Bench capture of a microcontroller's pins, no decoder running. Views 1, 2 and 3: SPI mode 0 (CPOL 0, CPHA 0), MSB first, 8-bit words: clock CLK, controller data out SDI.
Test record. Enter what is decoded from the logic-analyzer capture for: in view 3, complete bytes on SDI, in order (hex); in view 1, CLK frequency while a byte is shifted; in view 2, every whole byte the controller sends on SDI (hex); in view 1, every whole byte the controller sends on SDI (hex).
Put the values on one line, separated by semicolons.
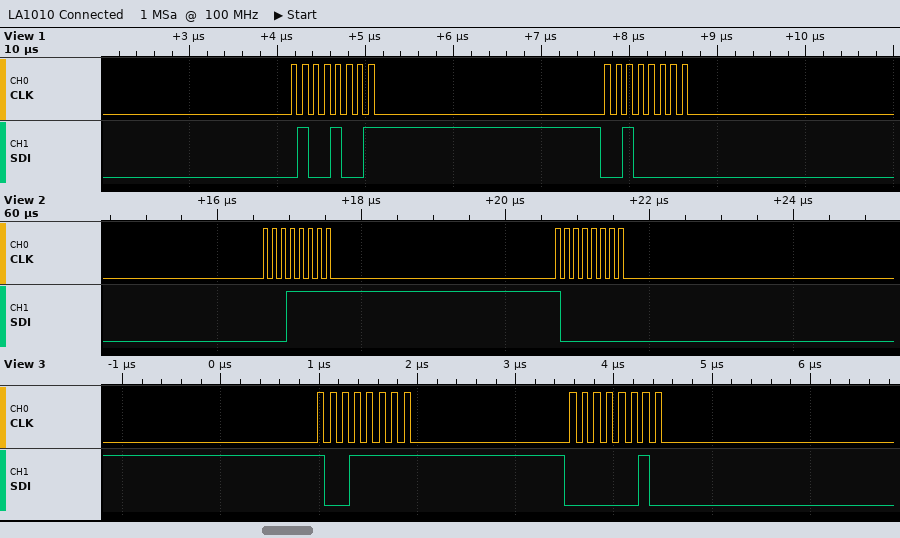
0x9F 0x02; 8 MHz; 1F 80; 49 20
